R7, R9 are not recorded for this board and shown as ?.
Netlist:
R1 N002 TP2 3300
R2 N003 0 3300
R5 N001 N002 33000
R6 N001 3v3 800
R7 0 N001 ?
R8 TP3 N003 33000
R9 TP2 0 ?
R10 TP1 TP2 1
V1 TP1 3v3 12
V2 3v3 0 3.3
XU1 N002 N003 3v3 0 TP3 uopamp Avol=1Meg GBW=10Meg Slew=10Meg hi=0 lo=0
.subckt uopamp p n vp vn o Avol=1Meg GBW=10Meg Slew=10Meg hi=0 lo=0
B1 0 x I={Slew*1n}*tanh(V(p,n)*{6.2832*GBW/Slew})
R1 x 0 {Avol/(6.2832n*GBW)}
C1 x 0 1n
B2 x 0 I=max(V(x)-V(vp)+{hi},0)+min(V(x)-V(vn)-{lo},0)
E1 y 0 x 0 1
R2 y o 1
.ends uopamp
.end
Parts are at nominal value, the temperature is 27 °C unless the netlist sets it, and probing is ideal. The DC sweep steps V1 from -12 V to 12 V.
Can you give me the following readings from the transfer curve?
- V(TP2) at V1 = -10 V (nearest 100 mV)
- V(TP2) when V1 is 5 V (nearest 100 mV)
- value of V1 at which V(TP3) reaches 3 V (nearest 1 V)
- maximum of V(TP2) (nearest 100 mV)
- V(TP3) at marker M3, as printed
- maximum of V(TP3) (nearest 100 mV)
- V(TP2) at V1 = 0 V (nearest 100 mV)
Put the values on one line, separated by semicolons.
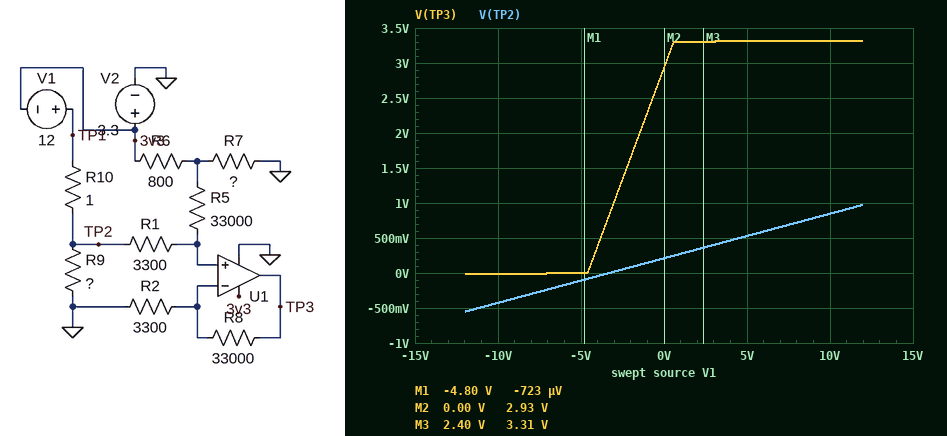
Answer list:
-400 mV; 500 mV; 0 V; 1.0 V; 3.31 V; 3.3 V; 200 mV
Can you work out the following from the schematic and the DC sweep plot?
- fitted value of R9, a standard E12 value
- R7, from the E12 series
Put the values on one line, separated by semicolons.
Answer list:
0.068 Ω; 270 Ω
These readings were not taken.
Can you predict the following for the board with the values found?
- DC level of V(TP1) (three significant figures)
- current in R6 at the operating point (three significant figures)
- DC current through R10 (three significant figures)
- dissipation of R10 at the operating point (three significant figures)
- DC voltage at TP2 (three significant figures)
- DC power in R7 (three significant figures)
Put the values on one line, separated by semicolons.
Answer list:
15.3 V; 3.08 mA; 14.3 A; 205 W; 974 mV; 2.57 mW
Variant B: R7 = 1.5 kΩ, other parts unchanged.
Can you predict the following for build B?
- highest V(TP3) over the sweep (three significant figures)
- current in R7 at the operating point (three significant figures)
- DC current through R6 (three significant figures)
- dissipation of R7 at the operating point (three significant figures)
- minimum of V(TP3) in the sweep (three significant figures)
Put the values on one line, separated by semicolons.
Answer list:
3.31 V; 1.42 mA; 1.46 mA; 3.04 mW; -9.60 mV
